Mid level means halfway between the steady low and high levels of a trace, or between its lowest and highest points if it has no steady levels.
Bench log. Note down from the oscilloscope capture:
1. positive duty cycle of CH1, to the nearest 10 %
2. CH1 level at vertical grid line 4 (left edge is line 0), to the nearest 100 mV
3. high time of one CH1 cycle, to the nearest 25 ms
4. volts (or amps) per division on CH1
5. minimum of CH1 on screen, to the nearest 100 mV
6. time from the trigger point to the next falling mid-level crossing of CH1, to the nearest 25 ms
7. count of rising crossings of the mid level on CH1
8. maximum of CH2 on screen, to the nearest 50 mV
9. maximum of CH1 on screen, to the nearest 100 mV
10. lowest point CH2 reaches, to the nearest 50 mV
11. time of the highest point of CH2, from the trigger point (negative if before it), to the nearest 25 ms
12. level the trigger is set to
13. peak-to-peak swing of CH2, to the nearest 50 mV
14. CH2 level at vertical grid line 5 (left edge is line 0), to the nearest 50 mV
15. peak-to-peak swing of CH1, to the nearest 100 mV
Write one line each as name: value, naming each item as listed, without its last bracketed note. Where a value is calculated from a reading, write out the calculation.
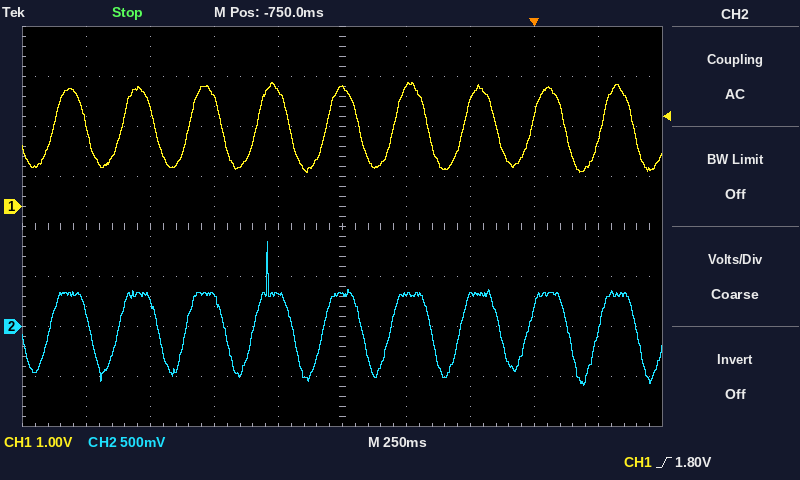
positive duty cycle of CH1, to the nearest 10 %: 50 %
CH1 level at vertical grid line 4 (left edge is line 0), to the nearest 100 mV: 2.3 V
high time of one CH1 cycle, to the nearest 25 ms: 125 ms
volts (or amps) per division on CH1: 1 V
minimum of CH1 on screen, to the nearest 100 mV: 700 mV
time from the trigger point to the next falling mid-level crossing of CH1, to the nearest 25 ms: 125 ms
count of rising crossings of the mid level on CH1: 9
maximum of CH2 on screen, to the nearest 50 mV: 850 mV
maximum of CH1 on screen, to the nearest 100 mV: 2.5 V
lowest point CH2 reaches, to the nearest 50 mV: -600 mV
time of the highest point of CH2, from the trigger point (negative if before it), to the nearest 25 ms: -1.050 s
level the trigger is set to: 1.80 V
peak-to-peak swing of CH2, to the nearest 50 mV: 850 mV − (-600 mV) = 1.45 V
CH2 level at vertical grid line 5 (left edge is line 0), to the nearest 50 mV: 300 mV
peak-to-peak swing of CH1, to the nearest 100 mV: 2.5 V − (700 mV) = 1.8 V
